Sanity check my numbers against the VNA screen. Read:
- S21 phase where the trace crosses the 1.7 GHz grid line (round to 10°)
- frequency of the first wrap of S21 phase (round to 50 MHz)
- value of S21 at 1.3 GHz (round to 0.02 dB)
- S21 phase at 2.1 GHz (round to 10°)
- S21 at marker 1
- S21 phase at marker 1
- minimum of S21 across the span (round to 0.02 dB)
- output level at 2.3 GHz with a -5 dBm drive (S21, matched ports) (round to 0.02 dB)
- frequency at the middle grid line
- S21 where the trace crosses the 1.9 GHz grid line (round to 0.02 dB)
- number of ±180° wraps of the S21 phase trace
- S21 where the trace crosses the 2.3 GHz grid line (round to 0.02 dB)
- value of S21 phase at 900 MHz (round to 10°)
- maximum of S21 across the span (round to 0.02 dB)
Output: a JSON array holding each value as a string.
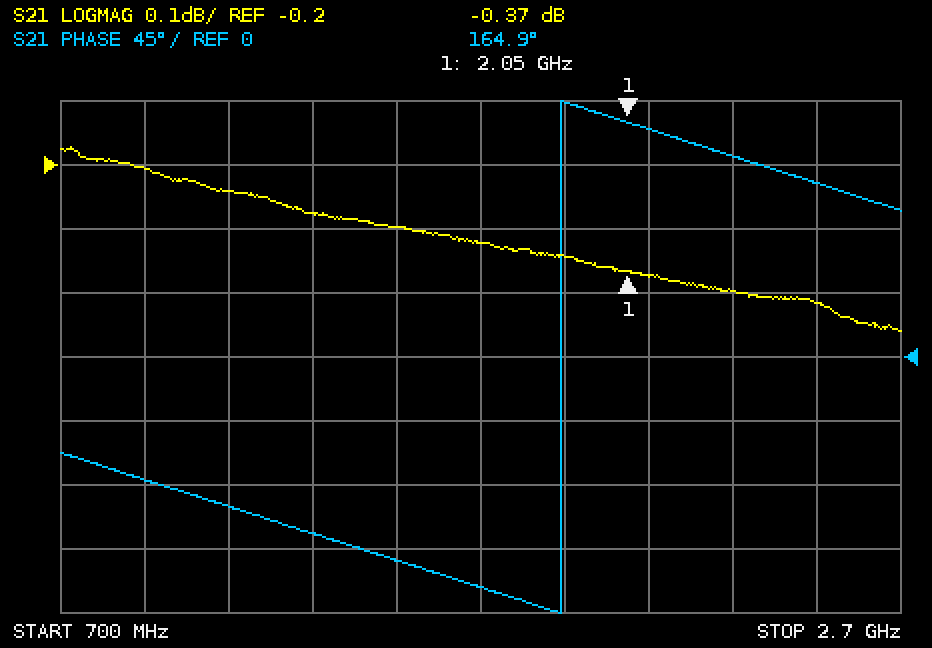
["-160°", "1.90 GHz", "-0.28 dB", "160°", "-0.37 dB", "164.9°", "-0.46 dB", "-5.40 dBm", "1.7 GHz", "-0.34 dB", "1", "-0.40 dB", "-90°", "-0.18 dB"]
